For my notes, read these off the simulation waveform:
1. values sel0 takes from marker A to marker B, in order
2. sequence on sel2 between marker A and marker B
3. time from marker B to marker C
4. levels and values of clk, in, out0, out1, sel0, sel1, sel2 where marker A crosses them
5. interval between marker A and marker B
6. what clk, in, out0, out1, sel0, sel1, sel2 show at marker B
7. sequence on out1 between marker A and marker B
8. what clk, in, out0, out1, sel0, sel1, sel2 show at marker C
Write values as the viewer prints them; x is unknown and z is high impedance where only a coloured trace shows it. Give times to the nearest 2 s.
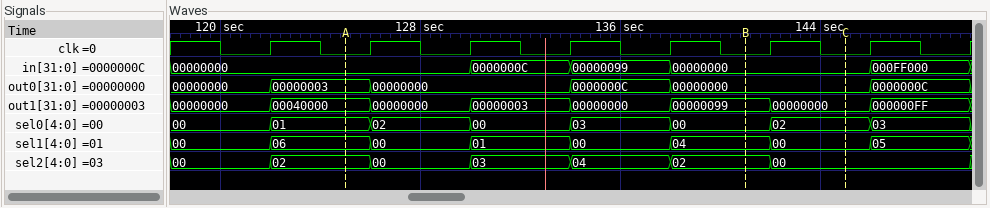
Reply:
01, 02, 00, 03, 00
02, 00, 03, 04, 02
4 s
clk=0, in=00000000, out0=00000003, out1=00040000, sel0=01, sel1=06, sel2=02
16 s
clk=0, in=00000000, out0=00000000, out1=00000099, sel0=00, sel1=04, sel2=02
00040000, 00000000, 00000003, 00000000, 00000099
clk=0, in=00000000, out0=00000000, out1=00000000, sel0=02, sel1=00, sel2=00
